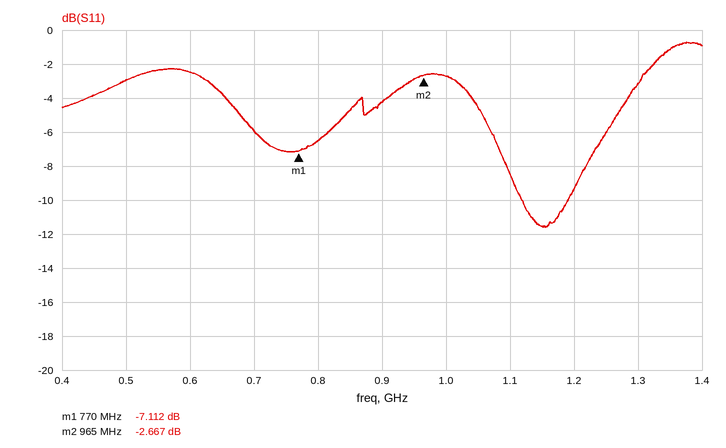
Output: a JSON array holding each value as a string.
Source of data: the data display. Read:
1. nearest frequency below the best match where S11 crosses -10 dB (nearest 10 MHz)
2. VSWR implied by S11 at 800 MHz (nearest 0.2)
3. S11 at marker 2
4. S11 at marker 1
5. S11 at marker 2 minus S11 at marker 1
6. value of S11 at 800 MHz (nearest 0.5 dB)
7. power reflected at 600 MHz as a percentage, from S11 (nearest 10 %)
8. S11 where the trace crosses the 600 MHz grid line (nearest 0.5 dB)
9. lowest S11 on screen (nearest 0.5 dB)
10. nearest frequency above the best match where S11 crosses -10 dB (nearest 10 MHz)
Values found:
["1.12 GHz", "2.8", "-2.667 dB", "-7.112 dB", "4.445 dB", "-6.5 dB", "60 %", "-2.5 dB", "-11.5 dB", "1.19 GHz"]
